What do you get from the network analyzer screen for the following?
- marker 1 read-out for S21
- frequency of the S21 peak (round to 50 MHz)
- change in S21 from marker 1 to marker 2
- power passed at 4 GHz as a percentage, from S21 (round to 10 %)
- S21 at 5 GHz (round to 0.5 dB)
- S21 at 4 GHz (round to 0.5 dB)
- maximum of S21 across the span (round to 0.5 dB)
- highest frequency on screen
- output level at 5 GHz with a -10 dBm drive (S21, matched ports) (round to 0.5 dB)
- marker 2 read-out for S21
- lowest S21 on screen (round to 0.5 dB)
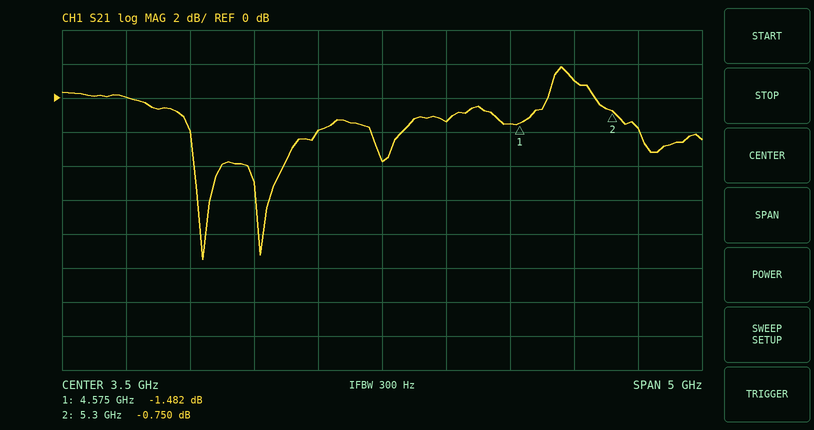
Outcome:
-1.482 dB
4.90 GHz
0.732 dB
70 %
1.0 dB
-1.5 dB
2.0 dB
6 GHz
-9.0 dBm
-0.750 dB
-9.5 dB
